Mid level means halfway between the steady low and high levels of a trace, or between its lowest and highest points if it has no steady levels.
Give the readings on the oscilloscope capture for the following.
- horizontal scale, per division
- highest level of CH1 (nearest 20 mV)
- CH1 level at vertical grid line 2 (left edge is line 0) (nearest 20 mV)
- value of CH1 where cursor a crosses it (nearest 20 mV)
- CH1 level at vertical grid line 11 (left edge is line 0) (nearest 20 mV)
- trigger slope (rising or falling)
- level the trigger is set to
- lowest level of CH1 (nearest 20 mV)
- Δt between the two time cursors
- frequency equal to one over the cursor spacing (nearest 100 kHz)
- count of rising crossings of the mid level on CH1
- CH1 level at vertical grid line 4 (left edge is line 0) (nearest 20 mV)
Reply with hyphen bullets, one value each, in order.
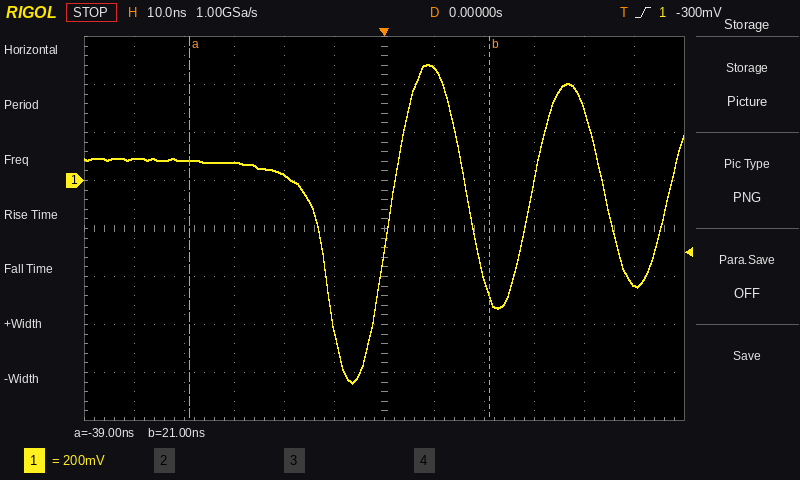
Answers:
- 10 ns
- 480 mV
- 80 mV
- 80 mV
- -440 mV
- rising
- -300 mV
- -840 mV
- 60 ns
- 16.7 MHz
- 3
- 20 mV
